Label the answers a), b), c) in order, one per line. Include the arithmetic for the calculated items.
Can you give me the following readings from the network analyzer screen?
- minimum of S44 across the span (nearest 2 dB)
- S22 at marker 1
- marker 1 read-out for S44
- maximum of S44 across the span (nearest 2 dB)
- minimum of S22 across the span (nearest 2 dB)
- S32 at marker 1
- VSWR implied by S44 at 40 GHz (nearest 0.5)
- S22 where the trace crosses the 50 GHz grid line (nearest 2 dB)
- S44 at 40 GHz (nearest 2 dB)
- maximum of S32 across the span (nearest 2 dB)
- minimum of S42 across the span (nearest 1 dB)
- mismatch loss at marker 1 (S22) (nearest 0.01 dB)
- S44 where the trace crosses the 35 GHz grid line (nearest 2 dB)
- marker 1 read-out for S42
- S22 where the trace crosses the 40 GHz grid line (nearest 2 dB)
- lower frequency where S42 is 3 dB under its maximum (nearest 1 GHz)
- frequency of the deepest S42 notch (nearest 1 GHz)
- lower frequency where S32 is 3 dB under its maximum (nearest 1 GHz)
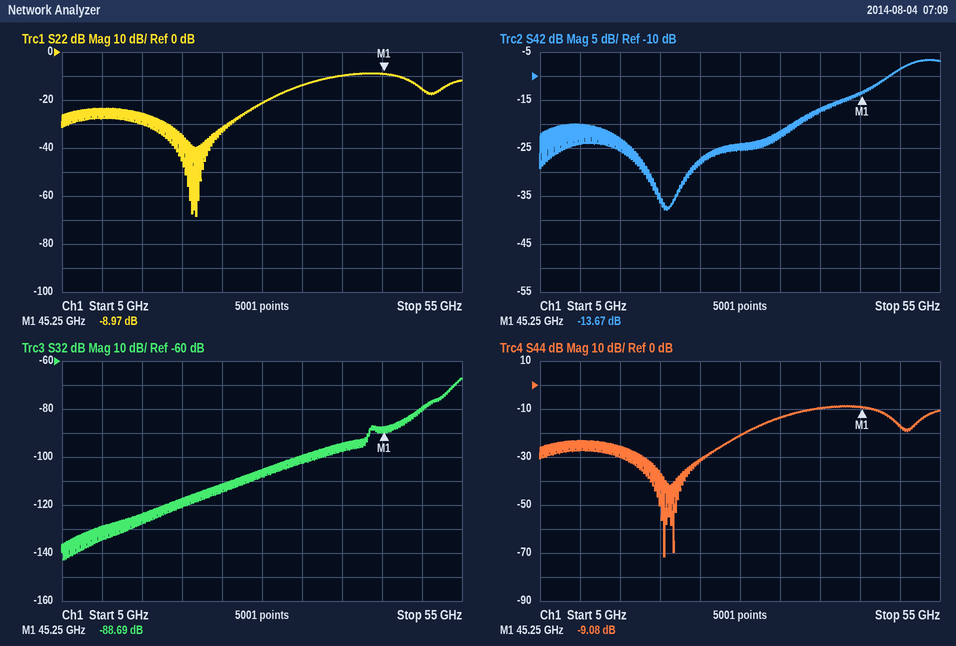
a) -72 dB
b) -8.97 dB
c) -9.08 dB
d) -8 dB
e) -68 dB
f) -88.69 dB
g) |Γ| = 10^(-10/20) = 0.3162; VSWR = (1 + 0.3162)/(1 − 0.3162) ≈ 1.92, so 2.0 to the nearest 0.5
h) -16 dB
i) -10 dB
j) -68 dB
k) -38 dB
l) −10 log10(1 − 10^(-8.97/10)) ≈ 0.59 dB
m) -14 dB
n) -13.67 dB
o) -10 dB
p) 49 GHz
q) 21 GHz
r) 54 GHz
